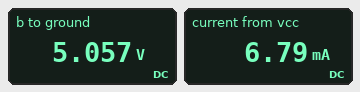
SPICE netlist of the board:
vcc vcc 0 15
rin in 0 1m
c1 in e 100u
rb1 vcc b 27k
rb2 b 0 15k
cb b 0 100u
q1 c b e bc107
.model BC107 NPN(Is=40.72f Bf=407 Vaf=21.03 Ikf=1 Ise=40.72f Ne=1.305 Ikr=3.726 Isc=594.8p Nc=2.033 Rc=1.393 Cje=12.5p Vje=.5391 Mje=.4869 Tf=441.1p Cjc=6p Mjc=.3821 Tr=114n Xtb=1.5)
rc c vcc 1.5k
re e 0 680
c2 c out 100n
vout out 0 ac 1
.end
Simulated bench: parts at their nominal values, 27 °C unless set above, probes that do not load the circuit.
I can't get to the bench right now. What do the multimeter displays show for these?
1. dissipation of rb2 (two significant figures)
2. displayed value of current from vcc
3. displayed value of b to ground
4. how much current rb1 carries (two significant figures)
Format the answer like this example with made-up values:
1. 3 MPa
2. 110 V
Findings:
1. 1.7 mW
2. 6.79 mA
3. 5.057 V
4. 370 µA
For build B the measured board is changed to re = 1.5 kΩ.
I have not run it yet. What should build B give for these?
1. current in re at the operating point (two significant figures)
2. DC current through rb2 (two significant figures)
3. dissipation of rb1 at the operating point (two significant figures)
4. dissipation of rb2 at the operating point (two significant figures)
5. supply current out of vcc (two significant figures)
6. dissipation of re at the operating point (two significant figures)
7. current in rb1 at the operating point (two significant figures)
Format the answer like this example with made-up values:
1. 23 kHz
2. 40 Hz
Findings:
1. 3.1 mA
2. 350 µA
3. 3.5 mW
4. 1.8 mW
5. 3.4 mA
6. 14 mW
7. 360 µA
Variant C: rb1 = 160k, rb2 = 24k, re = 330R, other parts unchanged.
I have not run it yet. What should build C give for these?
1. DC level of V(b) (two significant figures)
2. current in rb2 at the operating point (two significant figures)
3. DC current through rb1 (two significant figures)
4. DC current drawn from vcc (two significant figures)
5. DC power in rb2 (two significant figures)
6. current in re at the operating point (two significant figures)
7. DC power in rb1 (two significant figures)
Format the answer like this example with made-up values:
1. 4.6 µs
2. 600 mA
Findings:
1. 1.7 V
2. 71 µA
3. 83 µA
4. 3.3 mA
5. 120 µW
6. 3.2 mA
7. 1.1 mW
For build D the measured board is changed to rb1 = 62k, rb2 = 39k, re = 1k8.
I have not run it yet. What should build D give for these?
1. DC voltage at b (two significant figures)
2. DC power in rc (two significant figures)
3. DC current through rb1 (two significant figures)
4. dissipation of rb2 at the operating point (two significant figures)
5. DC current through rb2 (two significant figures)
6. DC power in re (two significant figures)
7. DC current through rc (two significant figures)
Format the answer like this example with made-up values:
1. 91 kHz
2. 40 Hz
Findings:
1. 5.5 V
2. 11 mW
3. 150 µA
4. 780 µW
5. 140 µA
6. 13 mW
7. 2.7 mA
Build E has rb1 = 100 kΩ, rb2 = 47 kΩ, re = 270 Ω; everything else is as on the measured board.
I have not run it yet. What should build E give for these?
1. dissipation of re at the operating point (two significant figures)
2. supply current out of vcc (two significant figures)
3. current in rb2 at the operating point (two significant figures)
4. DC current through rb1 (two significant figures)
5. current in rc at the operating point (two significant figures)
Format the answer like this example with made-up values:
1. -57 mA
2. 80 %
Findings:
1. 19 mW
2. 8.5 mA
3. 63 µA
4. 120 µA
5. 8.4 mA
